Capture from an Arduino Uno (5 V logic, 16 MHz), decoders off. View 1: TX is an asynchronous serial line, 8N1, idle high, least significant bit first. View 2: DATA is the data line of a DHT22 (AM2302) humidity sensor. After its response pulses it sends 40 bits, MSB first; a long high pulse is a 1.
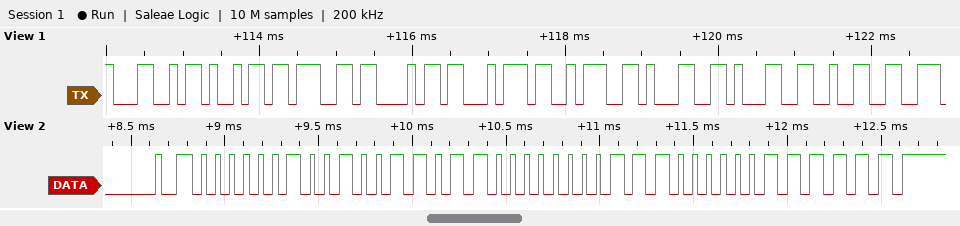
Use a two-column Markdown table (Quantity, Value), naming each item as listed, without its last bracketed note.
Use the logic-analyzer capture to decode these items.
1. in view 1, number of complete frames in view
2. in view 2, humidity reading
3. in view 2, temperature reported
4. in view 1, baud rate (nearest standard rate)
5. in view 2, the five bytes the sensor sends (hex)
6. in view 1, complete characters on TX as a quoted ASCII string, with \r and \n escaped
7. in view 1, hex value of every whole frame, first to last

| Quantity | Value |
|---|---|
| in view 1, number of complete frames in view | 9 |
| in view 2, humidity reading | 58.9 % |
| in view 2, temperature reported | -11.2 °C |
| in view 1, baud rate | 9600 baud |
| in view 2, the five bytes the sensor sends | 02 4D 80 70 3F |
| in view 1, complete characters on TX as a quoted ASCII string, with \r and \n escaped | "Light:112" |
| in view 1, hex value of every whole frame, first to last | 4C 69 67 68 74 3A 31 31 32 |
